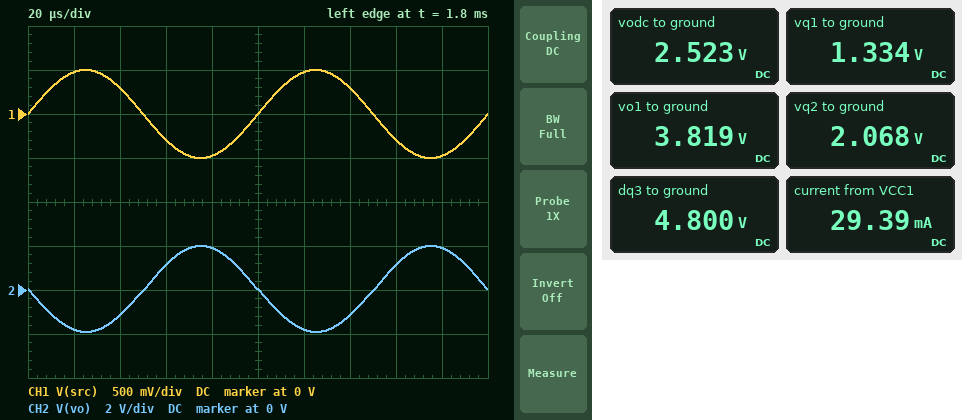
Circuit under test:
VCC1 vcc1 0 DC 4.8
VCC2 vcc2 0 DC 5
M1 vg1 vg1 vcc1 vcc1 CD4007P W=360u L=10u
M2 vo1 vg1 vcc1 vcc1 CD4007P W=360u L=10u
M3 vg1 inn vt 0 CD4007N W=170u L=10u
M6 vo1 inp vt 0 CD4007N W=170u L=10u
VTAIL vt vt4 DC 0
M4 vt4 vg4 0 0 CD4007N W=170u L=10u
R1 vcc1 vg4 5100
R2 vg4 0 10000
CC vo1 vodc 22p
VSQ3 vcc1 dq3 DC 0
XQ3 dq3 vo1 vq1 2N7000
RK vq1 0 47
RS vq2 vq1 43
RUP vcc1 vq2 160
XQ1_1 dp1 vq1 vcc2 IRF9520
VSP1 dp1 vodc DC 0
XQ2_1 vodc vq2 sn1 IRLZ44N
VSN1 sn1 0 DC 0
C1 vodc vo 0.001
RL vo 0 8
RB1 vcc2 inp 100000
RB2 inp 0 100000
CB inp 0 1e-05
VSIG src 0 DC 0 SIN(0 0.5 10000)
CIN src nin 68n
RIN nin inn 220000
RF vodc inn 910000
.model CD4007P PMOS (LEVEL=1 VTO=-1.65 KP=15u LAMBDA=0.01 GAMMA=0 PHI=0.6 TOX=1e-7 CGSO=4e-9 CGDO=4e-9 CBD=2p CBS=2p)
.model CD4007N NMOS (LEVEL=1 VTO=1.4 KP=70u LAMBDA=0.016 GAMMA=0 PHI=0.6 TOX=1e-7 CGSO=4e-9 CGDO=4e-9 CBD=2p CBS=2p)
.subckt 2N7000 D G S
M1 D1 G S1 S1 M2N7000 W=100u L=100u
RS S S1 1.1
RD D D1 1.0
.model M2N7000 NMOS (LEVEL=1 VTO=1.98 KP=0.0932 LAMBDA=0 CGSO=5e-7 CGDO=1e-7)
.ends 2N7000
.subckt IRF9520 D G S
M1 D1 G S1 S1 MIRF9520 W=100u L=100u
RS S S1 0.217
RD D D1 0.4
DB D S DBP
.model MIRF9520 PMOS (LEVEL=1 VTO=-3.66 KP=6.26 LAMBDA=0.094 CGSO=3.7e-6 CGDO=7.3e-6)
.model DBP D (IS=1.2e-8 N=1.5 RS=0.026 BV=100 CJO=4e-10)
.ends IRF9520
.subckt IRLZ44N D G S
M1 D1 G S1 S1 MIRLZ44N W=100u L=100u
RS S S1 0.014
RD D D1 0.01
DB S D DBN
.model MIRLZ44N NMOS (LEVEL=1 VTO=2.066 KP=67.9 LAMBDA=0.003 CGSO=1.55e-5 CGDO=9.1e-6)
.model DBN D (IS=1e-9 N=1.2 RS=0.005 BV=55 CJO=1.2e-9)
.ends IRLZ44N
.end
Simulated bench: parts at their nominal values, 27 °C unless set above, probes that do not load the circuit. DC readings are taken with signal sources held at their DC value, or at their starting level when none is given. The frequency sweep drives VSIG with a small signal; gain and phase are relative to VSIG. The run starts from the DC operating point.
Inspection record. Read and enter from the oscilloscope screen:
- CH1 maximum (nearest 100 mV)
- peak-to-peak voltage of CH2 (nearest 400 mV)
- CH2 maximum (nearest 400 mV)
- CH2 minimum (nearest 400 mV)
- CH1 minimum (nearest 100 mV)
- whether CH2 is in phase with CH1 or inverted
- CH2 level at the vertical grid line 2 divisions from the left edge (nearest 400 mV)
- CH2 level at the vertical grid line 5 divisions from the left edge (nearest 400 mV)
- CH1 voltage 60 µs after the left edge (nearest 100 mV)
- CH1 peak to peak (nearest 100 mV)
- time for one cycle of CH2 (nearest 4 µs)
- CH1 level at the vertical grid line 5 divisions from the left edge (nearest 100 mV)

500 mV
4.0 V
2.0 V
-2.0 V
-500 mV
inverted
-1.2 V
0 V
-300 mV
1.0 V
100 µs
0 V
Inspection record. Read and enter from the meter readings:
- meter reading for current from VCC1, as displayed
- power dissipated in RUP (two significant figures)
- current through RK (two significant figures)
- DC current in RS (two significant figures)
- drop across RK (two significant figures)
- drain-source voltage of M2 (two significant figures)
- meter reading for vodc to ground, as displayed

29.39 mA
47 mW
28 mA
17 mA
1.3 V
-980 mV
2.523 V
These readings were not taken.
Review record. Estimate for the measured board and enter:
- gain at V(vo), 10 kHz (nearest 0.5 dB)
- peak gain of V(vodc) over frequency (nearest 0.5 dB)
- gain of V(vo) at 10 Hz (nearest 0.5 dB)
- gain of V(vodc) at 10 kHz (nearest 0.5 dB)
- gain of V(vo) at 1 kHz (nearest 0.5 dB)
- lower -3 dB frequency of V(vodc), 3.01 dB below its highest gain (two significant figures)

7.5 dB
9.5 dB
2.0 dB
7.5 dB
7.5 dB
6.1 Hz
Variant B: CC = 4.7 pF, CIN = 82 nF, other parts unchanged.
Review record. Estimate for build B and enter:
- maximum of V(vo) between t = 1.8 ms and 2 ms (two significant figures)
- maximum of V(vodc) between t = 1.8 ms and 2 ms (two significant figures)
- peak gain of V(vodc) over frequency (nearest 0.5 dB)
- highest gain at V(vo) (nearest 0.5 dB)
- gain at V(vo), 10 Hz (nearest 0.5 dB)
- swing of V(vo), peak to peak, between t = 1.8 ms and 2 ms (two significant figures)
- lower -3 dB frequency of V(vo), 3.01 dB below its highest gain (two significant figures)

2.2 V
4.7 V
10.0 dB
9.5 dB
3.0 dB
4.1 V
20 Hz
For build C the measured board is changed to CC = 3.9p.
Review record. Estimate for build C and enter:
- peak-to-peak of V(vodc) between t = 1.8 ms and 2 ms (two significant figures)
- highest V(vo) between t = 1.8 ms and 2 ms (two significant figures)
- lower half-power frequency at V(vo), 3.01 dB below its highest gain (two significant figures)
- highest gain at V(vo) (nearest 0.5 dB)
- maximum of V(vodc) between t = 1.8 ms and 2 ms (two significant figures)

4.1 V
2.2 V
22 Hz
9.5 dB
4.7 V
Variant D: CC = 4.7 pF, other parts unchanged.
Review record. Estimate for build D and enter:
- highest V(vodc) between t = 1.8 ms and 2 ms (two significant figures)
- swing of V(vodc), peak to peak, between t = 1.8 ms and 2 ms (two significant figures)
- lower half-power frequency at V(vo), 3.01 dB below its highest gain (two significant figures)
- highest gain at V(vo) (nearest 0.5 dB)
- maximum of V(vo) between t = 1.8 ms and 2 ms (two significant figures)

4.7 V
4.1 V
21 Hz
9.5 dB
2.2 V
